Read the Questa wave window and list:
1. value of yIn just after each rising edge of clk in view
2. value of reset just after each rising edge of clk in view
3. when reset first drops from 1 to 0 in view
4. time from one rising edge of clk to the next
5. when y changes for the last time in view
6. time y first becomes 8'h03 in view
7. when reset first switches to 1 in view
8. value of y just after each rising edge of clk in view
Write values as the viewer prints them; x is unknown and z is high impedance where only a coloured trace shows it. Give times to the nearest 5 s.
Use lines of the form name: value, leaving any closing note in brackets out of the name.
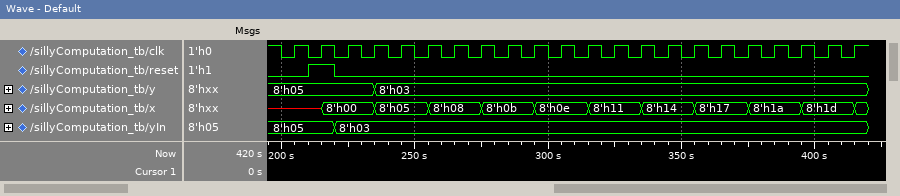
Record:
value of yIn just after each rising edge of clk in view: 8'h05, 8'h05, 8'h03, 8'h03, 8'h03, 8'h03, 8'h03, 8'h03, 8'h03, 8'h03, 8'h03, 8'h03, 8'h03, 8'h03, 8'h03, 8'h03, 8'h03, 8'h03, 8'h03, 8'h03, 8'h03, 8'h03
value of reset just after each rising edge of clk in view: 0 1 0 0 0 0 0 0 0 0 0 0 0 0 0 0 0 0 0 0 0 0
when reset first drops from 1 to 0 in view: 220 s
time from one rising edge of clk to the next: 10 s
when y changes for the last time in view: 235 s
time y first becomes 8'h03 in view: 235 s
when reset first switches to 1 in view: 210 s
value of y just after each rising edge of clk in view: 8'h05, 8'h05, 8'h05, 8'h03, 8'h03, 8'h03, 8'h03, 8'h03, 8'h03, 8'h03, 8'h03, 8'h03, 8'h03, 8'h03, 8'h03, 8'h03, 8'h03, 8'h03, 8'h03, 8'h03, 8'h03, 8'h03
